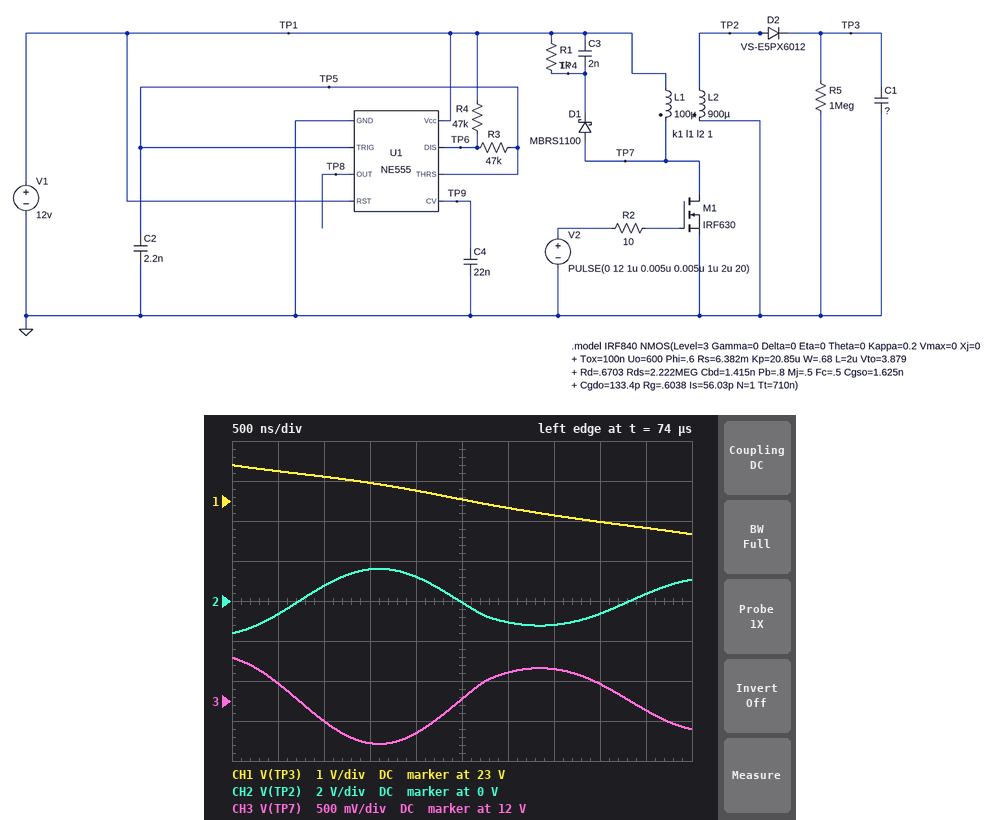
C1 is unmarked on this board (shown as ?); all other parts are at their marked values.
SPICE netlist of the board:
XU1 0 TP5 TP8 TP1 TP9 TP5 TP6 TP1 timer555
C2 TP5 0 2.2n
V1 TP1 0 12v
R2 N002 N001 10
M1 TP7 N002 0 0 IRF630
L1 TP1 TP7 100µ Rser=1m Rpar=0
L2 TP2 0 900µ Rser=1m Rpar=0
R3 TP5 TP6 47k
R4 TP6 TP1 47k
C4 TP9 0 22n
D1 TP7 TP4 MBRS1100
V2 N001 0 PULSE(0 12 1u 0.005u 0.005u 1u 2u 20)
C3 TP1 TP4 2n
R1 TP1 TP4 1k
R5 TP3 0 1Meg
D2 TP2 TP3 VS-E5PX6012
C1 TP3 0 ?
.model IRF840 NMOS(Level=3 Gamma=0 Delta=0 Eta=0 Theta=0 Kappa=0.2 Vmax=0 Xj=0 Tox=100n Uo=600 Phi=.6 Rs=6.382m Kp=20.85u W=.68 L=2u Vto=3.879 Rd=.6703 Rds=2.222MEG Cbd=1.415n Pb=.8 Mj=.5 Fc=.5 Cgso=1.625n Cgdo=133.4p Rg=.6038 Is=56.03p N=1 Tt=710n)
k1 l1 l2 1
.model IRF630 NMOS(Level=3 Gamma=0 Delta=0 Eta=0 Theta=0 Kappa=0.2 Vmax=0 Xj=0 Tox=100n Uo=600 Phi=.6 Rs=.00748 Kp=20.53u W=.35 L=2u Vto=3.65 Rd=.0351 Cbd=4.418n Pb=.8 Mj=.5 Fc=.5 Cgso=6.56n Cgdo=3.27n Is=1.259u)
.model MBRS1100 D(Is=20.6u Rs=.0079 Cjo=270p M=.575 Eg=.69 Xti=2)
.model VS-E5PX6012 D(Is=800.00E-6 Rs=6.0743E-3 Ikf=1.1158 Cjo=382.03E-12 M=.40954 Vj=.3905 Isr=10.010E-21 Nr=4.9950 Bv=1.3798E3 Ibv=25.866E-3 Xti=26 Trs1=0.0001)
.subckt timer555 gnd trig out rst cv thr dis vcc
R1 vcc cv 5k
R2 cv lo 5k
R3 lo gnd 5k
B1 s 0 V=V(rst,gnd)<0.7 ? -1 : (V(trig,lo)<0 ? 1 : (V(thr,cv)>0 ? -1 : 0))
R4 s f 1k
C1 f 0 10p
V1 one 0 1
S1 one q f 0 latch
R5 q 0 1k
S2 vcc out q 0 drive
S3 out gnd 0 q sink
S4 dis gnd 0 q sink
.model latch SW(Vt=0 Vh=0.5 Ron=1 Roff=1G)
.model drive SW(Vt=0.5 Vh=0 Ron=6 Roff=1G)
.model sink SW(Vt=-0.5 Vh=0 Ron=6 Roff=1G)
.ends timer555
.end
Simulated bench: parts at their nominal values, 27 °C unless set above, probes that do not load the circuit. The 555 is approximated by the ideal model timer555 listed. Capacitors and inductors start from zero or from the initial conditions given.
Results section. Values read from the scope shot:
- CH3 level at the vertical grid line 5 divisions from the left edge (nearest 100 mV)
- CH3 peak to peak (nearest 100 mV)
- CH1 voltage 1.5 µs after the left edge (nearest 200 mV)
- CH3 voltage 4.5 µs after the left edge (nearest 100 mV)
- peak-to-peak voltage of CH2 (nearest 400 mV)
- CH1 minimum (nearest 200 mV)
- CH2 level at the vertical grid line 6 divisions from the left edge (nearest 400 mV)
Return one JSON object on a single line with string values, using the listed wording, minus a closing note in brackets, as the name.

{"CH3 level at the vertical grid line 5 divisions from the left edge": "12.0 V", "CH3 peak to peak": "1.1 V", "CH1 voltage 1.5 µs after the left edge": "23.4 V", "CH3 voltage 4.5 µs after the left edge": "11.9 V", "peak-to-peak voltage of CH2": "3.2 V", "CH1 minimum": "22.2 V", "CH2 level at the vertical grid line 6 divisions from the left edge": "-1.2 V"}
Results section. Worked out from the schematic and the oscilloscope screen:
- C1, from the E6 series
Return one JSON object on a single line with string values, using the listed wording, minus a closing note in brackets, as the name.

{"C1, from the E6 series": "2.2 nF"}
